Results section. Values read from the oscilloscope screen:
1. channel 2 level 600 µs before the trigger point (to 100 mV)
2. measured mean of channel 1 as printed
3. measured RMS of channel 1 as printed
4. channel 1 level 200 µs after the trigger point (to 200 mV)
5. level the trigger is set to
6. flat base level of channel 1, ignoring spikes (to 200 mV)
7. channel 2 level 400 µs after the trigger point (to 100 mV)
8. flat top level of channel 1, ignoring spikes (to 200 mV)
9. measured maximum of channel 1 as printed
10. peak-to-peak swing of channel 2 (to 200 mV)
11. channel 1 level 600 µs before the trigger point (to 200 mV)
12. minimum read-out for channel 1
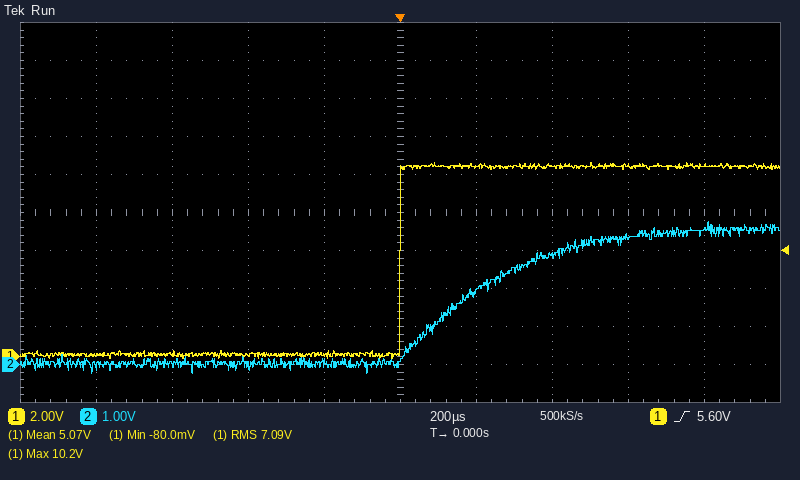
0.0 V
5.07 V
7.09 V
10.0 V
5.60 V
200 mV
2.9 V
10.0 V
10.2 V
4.0 V
200 mV
-80.0 mV
